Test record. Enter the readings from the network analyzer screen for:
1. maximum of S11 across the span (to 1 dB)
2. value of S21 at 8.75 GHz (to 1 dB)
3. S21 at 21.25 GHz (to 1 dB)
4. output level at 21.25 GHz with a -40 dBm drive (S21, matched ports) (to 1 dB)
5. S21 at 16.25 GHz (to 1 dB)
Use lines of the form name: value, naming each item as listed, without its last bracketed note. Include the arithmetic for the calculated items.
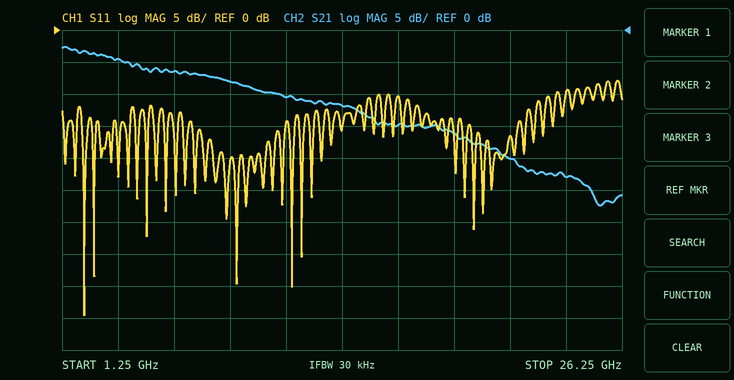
maximum of S11 across the span: -8 dB
value of S21 at 8.75 GHz: -8 dB
S21 at 21.25 GHz: -20 dB
output level at 21.25 GHz with a -40 dBm drive (S21, matched ports): -40 dBm + (-20 dB) = -60 dBm
S21 at 16.25 GHz: -15 dB
